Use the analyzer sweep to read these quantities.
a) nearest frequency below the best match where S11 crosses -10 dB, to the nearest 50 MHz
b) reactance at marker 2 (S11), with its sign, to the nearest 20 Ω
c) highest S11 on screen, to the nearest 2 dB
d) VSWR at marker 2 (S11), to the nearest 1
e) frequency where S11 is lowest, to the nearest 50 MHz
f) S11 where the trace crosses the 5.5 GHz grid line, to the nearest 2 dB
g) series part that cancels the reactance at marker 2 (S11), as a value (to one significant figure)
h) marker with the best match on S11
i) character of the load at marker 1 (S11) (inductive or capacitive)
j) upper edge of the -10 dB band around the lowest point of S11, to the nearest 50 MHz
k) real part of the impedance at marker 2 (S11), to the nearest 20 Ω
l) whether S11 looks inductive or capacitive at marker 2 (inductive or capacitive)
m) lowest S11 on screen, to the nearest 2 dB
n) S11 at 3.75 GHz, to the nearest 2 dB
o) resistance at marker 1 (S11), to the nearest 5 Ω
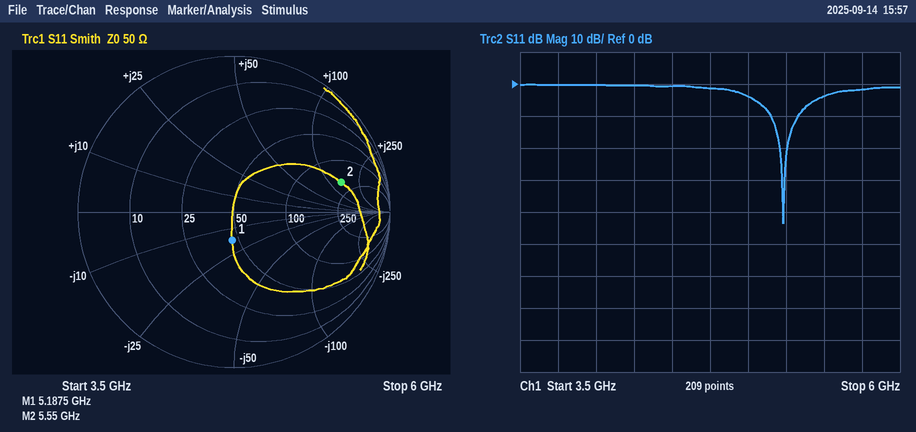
5.15 GHz
+140 Ω
0 dB
6
5.25 GHz
-4 dB
200 fF
marker 1
capacitive
5.35 GHz
180 Ω
inductive
-44 dB
0 dB
45 Ω
